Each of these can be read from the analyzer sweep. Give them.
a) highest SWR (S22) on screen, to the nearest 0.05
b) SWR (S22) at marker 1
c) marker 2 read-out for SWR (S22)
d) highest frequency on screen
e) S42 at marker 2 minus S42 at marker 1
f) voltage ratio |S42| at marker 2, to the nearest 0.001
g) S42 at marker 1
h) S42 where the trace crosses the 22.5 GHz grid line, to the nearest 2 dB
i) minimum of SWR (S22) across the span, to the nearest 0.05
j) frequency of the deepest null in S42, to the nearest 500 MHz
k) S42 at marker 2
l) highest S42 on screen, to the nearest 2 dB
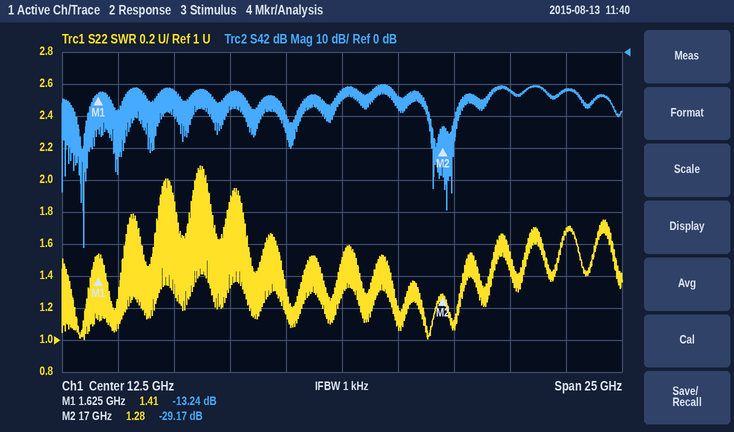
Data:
2.10
1.41
1.28
25 GHz
-15.93 dB
0.035
-13.24 dB
-12 dB
1.00
1.0 GHz
-29.17 dB
-10 dB
